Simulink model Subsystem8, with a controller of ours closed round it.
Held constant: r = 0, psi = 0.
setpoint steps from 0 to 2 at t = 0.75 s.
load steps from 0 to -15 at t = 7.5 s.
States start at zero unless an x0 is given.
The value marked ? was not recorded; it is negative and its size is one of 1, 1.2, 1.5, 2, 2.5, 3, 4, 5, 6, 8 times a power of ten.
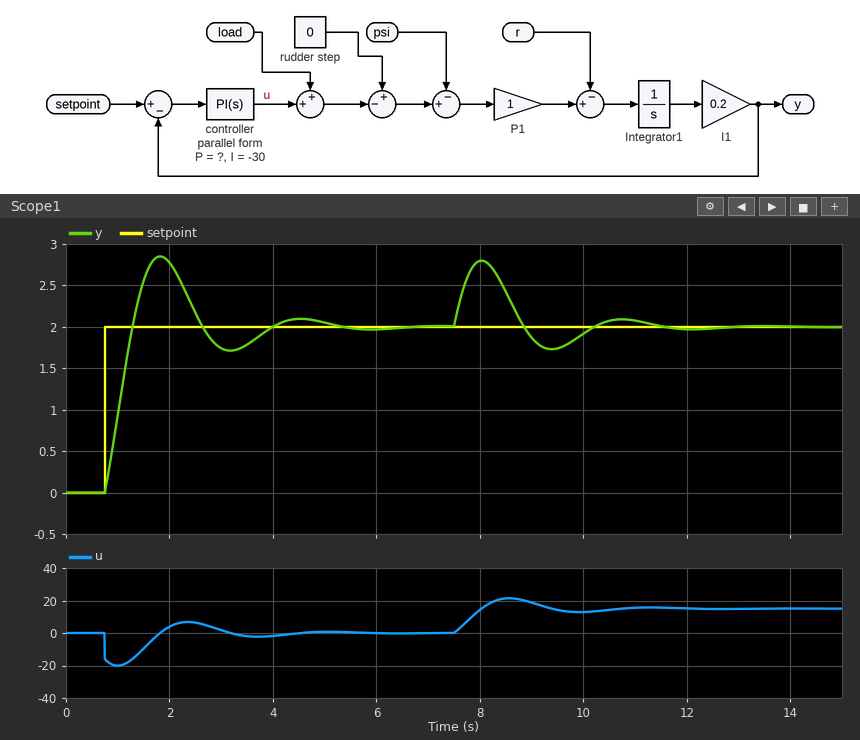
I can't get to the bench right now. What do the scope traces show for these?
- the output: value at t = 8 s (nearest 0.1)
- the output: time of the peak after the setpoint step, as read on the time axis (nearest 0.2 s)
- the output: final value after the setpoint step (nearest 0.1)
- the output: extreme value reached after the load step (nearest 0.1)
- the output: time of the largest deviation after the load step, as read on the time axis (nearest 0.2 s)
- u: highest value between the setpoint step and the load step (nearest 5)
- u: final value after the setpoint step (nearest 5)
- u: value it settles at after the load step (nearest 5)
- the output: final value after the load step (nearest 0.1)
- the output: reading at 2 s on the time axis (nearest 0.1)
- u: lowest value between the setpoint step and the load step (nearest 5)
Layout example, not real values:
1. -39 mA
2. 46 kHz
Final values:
1. 2.8
2. 1.8 s
3. 2.0
4. 2.8
5. 8.0 s
6. 5
7. 0
8. 15
9. 2.0
10. 2.8
11. -20
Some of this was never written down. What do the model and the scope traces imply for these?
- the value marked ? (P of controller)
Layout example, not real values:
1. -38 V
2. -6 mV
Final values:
1. -8
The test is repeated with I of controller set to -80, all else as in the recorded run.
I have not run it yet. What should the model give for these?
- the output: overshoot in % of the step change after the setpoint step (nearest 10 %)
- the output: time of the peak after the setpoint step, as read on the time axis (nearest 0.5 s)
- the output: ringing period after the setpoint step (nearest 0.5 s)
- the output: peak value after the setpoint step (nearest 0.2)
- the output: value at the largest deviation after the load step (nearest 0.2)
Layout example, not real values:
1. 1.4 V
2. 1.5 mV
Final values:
1. 60 %
2. 1.5 s
3. 1.5 s
4. 3.2
5. 2.6
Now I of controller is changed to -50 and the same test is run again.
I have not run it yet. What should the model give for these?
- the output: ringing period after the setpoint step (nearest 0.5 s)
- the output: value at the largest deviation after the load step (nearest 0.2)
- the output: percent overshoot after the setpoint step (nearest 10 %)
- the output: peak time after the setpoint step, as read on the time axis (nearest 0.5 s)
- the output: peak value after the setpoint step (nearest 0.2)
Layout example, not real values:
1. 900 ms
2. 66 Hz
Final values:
1. 2.0 s
2. 2.6
3. 50 %
4. 1.5 s
5. 3.0
